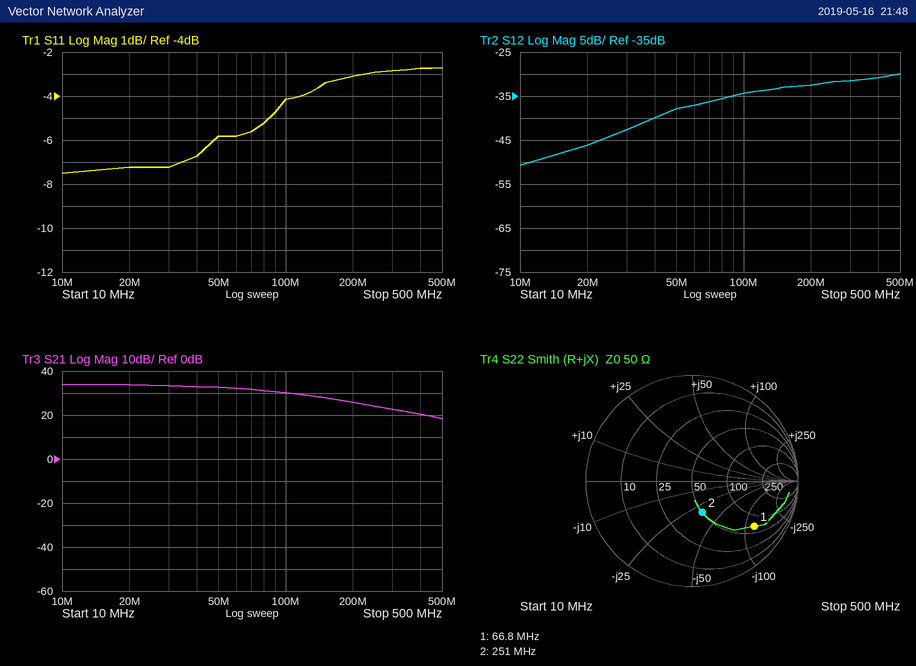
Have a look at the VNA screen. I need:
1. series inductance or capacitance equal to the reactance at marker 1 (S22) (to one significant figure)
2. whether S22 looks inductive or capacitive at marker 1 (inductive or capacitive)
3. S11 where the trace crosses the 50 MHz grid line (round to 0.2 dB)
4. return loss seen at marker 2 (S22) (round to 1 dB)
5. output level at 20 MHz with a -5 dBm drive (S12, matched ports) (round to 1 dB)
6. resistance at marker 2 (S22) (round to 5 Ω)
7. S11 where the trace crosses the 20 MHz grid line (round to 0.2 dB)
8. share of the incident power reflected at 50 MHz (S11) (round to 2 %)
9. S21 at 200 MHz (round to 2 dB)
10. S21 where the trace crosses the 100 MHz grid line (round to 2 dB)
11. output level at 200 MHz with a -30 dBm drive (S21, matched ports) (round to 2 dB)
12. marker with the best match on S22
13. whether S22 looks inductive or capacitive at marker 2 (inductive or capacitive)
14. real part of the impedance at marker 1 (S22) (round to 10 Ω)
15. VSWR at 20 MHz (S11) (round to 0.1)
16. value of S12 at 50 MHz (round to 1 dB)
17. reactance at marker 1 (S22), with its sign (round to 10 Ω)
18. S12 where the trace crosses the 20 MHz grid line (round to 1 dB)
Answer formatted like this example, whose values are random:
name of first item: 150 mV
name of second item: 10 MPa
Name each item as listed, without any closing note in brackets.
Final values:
series inductance or capacitance equal to the reactance at marker 1 (S22): 20 pF
whether S22 looks inductive or capacitive at marker 1: capacitive
S11 where the trace crosses the 50 MHz grid line: -5.8 dB
return loss seen at marker 2 (S22): 10 dB
output level at 20 MHz with a -5 dBm drive (S12, matched ports): -51 dBm
resistance at marker 2 (S22): 50 Ω
S11 where the trace crosses the 20 MHz grid line: -7.2 dB
share of the incident power reflected at 50 MHz (S11): 26 %
S21 at 200 MHz: 26 dB
S21 where the trace crosses the 100 MHz grid line: 30 dB
output level at 200 MHz with a -30 dBm drive (S21, matched ports): -4 dBm
marker with the best match on S22: marker 2
whether S22 looks inductive or capacitive at marker 2: capacitive
real part of the impedance at marker 1 (S22): 70 Ω
VSWR at 20 MHz (S11): 2.5
value of S12 at 50 MHz: -38 dB
reactance at marker 1 (S22), with its sign: -120 Ω
S12 where the trace crosses the 20 MHz grid line: -46 dB
